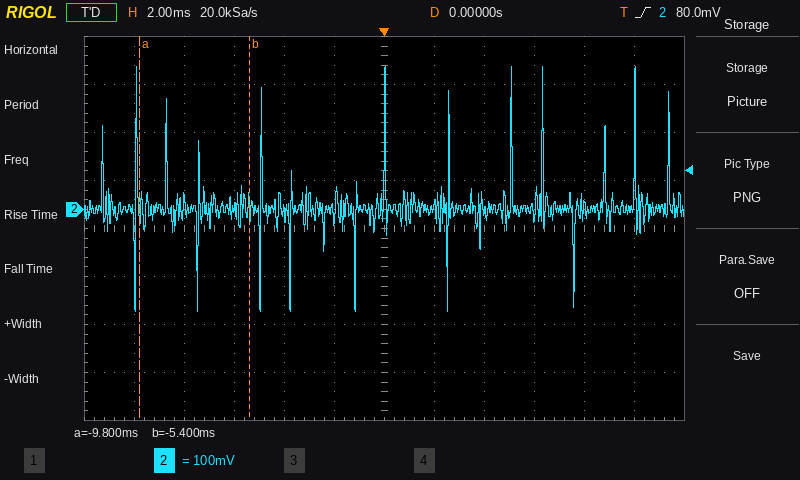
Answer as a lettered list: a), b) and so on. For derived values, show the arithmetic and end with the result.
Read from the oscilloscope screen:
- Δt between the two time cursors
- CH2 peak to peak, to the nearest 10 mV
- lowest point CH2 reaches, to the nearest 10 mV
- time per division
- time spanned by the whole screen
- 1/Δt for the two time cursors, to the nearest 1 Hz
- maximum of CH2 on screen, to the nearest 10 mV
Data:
a) -5.4 ms − (-9.8 ms) = 4.4 ms
b) 300 mV − (-210 mV) = 510 mV
c) -210 mV
d) 2 ms
e) 24 ms
f) 1 / 4.4 ms ≈ 227 Hz
g) 300 mV
